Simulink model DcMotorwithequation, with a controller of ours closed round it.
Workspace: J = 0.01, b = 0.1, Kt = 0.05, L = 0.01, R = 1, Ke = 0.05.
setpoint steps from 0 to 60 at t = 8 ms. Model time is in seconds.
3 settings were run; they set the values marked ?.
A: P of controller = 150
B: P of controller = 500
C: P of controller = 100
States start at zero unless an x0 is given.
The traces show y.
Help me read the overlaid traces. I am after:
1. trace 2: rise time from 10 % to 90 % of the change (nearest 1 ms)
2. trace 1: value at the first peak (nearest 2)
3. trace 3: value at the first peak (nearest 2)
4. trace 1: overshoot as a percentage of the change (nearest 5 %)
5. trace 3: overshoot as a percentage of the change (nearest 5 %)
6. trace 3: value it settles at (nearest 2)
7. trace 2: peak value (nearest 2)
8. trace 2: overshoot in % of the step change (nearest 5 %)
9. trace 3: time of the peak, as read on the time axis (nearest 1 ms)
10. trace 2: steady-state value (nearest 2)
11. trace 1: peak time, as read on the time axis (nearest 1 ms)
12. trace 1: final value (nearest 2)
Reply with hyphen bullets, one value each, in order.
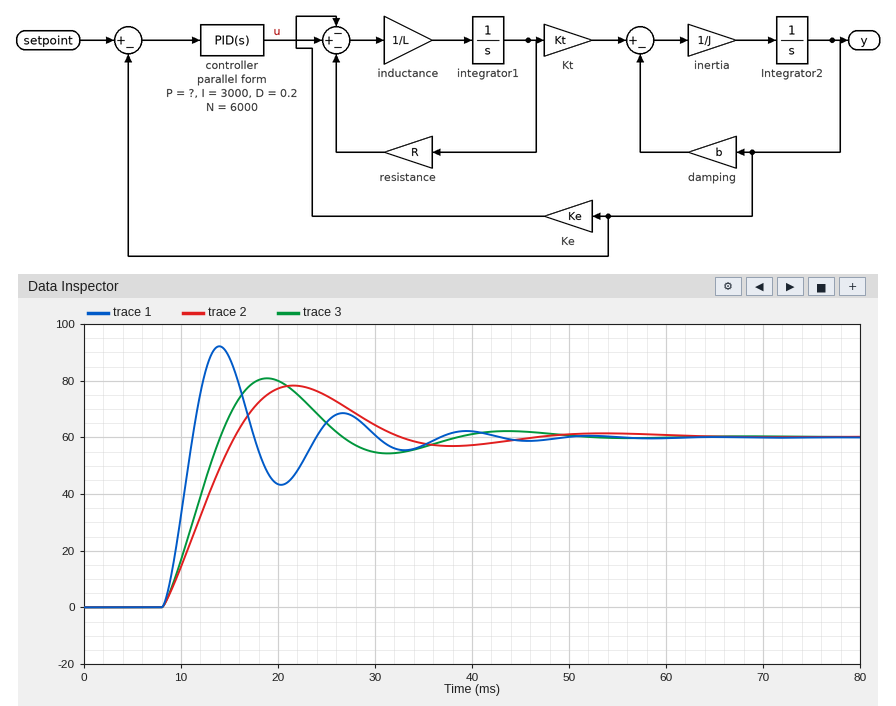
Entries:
- 6 ms
- 92
- 80
- 55 %
- 35 %
- 60
- 78
- 30 %
- 19 ms
- 60
- 14 ms
- 60
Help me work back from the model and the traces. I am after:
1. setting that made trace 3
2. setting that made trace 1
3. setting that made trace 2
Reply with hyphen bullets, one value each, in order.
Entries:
- A
- B
- C
